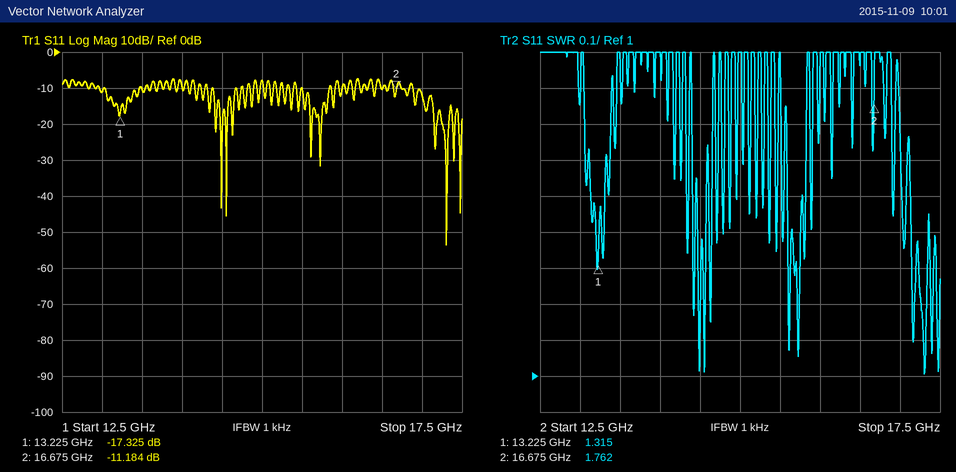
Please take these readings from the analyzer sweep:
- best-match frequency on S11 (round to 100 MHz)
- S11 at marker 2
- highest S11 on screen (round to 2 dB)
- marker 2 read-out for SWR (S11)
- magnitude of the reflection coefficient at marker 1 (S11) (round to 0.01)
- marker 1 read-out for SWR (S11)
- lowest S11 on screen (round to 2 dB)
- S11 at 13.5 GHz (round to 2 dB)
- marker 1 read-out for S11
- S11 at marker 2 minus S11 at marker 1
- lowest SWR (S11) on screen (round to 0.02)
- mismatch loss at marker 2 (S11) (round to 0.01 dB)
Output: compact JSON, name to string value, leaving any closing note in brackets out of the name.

{"best-match frequency on S11": "17.3 GHz", "S11 at marker 2": "-11.184 dB", "highest S11 on screen": "-8 dB", "marker 2 read-out for SWR": "1.762", "magnitude of the reflection coefficient at marker 1 (S11)": "0.14", "marker 1 read-out for SWR": "1.315", "lowest S11 on screen": "-54 dB", "S11 at 13.5 GHz": "-10 dB", "marker 1 read-out for S11": "-17.325 dB", "S11 at marker 2 minus S11 at marker 1": "6.141 dB", "lowest SWR (S11) on screen": "1.00", "mismatch loss at marker 2 (S11)": "0.34 dB"}
